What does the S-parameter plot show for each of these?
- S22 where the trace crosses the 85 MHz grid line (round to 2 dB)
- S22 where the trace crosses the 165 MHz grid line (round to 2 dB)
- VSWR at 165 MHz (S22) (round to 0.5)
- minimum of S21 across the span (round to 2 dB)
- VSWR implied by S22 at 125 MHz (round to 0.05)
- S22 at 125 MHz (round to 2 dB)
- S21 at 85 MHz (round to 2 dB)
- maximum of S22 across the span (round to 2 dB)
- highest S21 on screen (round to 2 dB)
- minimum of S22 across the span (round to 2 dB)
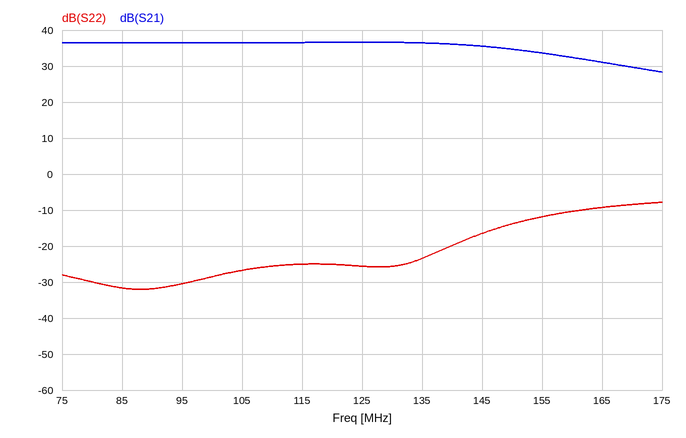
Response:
-32 dB
-10 dB
2.0
28 dB
1.10
-26 dB
36 dB
-8 dB
36 dB
-32 dB
